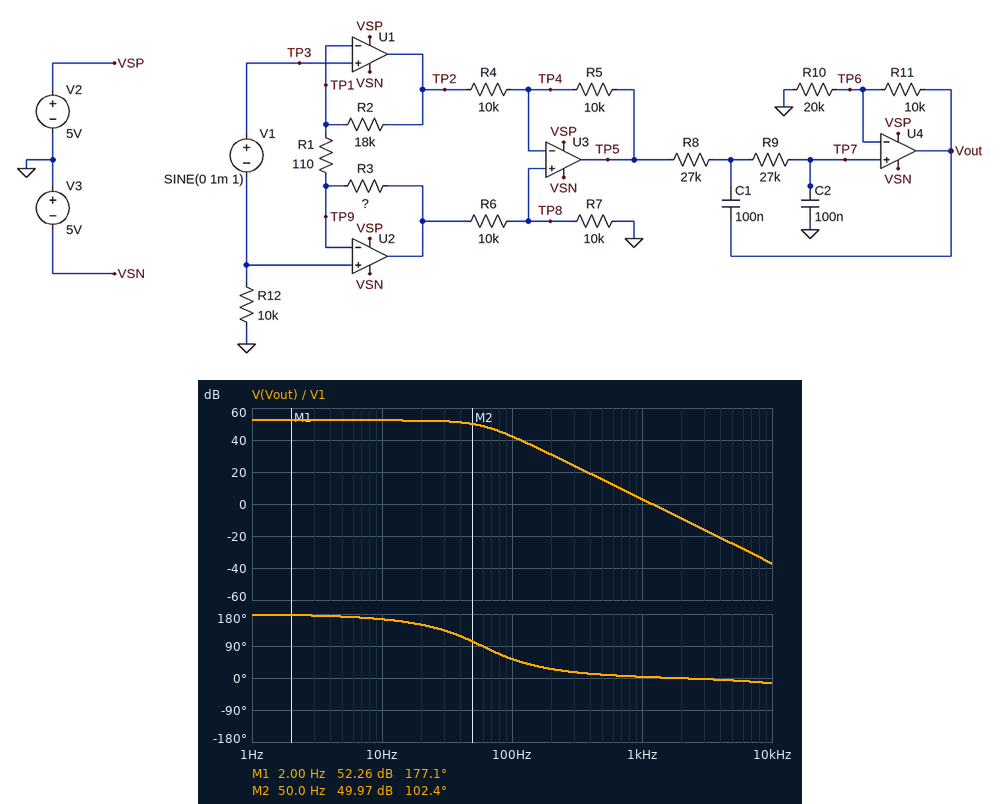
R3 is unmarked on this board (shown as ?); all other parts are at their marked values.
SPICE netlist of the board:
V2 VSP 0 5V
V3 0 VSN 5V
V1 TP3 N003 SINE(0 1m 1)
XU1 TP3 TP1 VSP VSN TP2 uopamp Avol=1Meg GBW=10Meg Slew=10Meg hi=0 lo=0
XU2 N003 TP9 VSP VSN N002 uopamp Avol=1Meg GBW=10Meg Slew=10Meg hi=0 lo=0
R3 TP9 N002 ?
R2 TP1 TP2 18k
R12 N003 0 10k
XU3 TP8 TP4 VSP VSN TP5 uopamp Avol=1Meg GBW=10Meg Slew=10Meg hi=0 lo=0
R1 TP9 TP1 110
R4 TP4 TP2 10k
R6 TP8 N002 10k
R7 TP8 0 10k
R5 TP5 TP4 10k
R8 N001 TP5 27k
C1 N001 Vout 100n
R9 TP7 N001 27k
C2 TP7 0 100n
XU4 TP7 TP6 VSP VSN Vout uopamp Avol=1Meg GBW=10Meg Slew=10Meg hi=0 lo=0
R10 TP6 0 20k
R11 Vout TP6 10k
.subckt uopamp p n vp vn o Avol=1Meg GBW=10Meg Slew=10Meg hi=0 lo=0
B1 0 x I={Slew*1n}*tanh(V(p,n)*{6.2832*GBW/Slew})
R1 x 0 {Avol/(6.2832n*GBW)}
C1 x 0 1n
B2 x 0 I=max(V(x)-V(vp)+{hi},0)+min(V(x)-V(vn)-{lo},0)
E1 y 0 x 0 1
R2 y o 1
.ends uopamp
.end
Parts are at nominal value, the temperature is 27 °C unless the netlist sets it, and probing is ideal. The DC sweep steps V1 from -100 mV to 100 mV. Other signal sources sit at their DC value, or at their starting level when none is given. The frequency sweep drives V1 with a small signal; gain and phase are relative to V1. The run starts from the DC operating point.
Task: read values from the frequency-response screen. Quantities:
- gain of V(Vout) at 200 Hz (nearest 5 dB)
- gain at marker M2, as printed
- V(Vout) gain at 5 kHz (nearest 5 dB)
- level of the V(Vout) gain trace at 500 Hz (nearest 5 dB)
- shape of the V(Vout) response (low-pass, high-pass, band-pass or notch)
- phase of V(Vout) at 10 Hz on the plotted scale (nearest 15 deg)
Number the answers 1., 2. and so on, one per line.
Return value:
1. 30 dB
2. 49.97 dB
3. -25 dB
4. 15 dB
5. low-pass
6. 165 deg
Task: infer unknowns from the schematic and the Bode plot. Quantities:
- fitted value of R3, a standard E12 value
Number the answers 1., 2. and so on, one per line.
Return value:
1. 12 kΩ
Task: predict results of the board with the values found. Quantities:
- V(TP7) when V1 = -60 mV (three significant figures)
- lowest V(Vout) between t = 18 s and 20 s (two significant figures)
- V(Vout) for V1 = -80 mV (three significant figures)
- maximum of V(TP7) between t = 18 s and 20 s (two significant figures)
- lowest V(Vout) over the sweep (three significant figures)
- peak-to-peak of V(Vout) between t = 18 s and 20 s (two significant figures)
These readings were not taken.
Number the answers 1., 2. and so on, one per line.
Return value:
1. 5.01 V
2. -410 mV
3. 5.01 V
4. 270 mV
5. -5.01 V
6. 820 mV
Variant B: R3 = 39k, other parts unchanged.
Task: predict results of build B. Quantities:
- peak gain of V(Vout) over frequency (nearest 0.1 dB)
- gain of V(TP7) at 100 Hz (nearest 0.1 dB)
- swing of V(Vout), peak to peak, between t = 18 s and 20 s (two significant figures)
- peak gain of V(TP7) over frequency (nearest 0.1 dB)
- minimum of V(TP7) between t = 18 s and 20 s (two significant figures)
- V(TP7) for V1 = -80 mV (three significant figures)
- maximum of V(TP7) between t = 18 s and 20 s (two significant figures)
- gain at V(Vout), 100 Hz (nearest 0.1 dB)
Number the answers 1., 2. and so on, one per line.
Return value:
1. 57.8 dB
2. 44.3 dB
3. 1.6 V
4. 54.3 dB
5. -520 mV
6. 5.01 V
7. 520 mV
8. 47.8 dB
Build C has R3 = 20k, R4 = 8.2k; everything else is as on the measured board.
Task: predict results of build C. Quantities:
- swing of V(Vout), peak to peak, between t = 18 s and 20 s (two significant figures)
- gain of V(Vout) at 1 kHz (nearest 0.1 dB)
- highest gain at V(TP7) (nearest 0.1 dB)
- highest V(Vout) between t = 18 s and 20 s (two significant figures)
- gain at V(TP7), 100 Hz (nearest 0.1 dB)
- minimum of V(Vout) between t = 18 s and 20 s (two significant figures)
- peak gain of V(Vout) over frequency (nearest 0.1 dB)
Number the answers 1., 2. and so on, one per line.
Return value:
1. 1.2 V
2. 6.4 dB
3. 52.1 dB
4. 600 mV
5. 42.1 dB
6. -600 mV
7. 55.6 dB
